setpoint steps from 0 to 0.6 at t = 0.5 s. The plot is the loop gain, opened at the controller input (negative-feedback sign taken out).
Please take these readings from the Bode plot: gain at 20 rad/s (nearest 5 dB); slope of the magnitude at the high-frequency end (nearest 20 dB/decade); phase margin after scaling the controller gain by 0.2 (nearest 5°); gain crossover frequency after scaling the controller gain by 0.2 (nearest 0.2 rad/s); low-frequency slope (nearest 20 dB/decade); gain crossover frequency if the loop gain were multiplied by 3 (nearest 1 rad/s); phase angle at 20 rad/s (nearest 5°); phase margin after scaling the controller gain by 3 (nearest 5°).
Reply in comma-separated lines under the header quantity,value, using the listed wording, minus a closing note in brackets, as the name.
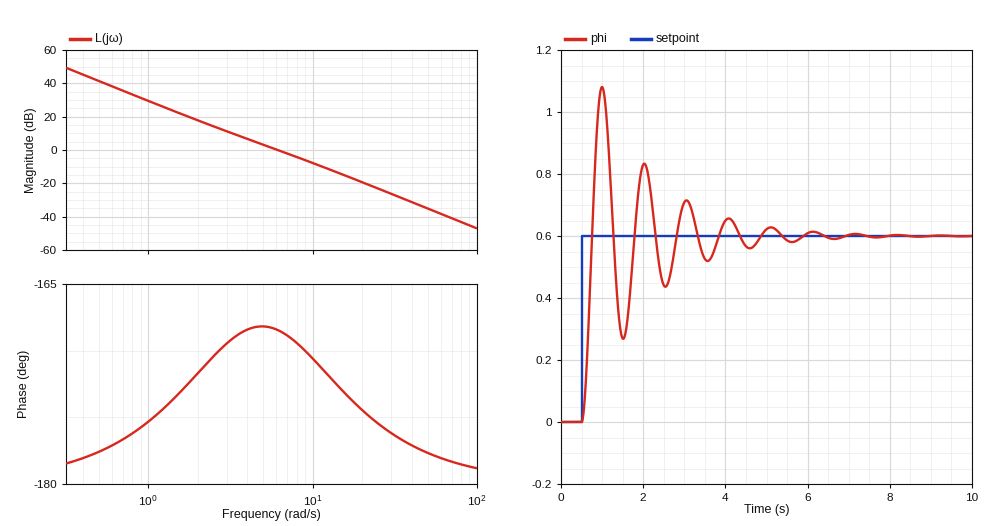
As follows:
quantity,value
gain at 20 rad/s,-20 dB
slope of the magnitude at the high-frequency end,-40 dB/decade
phase margin after scaling the controller gain by 0.2,10°
gain crossover frequency after scaling the controller gain by 0.2,2.6 rad/s
low-frequency slope,-40 dB/decade
gain crossover frequency if the loop gain were multiplied by 3,11 rad/s
phase angle at 20 rad/s,-175°
phase margin after scaling the controller gain by 3,10°
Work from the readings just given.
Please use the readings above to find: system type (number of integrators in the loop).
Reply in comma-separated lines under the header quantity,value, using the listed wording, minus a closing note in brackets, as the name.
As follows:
quantity,value
system type,2
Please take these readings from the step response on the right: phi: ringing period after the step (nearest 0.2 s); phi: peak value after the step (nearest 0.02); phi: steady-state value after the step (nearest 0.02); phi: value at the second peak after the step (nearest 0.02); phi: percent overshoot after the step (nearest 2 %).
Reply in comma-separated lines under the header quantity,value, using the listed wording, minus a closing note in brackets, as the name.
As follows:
quantity,value
phi: ringing period after the step,1.0 s
phi: peak value after the step,1.08
phi: steady-state value after the step,0.60
phi: value at the second peak after the step,0.84
phi: percent overshoot after the step,80 %
